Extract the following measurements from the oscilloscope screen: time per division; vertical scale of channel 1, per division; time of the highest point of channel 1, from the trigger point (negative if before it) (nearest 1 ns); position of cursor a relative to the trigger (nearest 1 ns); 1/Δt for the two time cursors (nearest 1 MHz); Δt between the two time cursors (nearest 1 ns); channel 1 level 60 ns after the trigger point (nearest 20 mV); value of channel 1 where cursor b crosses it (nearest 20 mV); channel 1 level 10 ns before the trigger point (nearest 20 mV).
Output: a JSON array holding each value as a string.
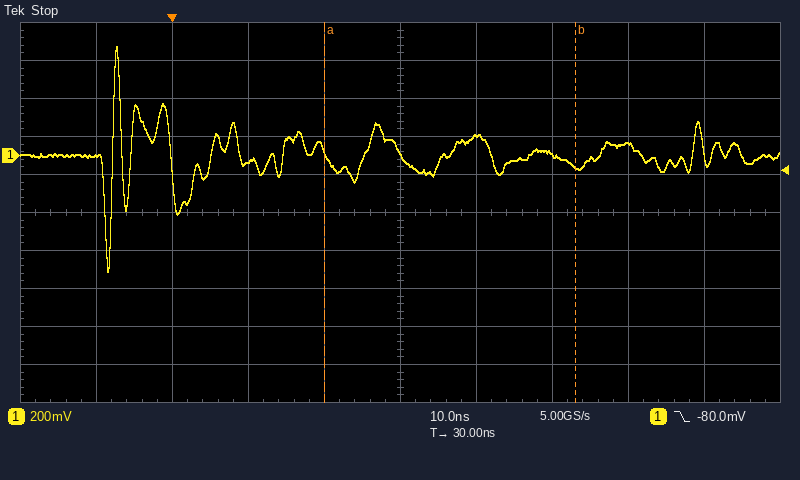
["10 ns", "200 mV", "-7 ns", "+20 ns", "30 MHz", "33 ns", "60 mV", "-60 mV", "0 mV"]
